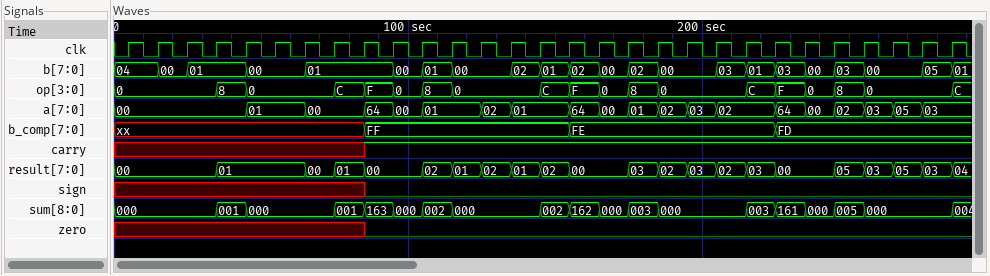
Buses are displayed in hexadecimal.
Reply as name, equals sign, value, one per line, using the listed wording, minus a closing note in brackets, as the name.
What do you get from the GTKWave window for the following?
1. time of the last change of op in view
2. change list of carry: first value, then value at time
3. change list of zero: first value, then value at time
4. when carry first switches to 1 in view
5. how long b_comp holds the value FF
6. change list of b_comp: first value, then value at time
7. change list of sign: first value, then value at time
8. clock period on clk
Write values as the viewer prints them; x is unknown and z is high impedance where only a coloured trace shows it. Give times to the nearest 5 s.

time of the last change of op in view = 285 s
change list of carry: first value, then value at time = x, 1 at 85 s
change list of zero: first value, then value at time = x, 0 at 85 s
when carry first switches to 1 in view = 85 s
how long b_comp holds the value FF = 70 s
change list of b_comp: first value, then value at time = xx, FF at 85 s, FE at 155 s, FD at 225 s
change list of sign: first value, then value at time = x, 0 at 85 s
clock period on clk = 10 s
